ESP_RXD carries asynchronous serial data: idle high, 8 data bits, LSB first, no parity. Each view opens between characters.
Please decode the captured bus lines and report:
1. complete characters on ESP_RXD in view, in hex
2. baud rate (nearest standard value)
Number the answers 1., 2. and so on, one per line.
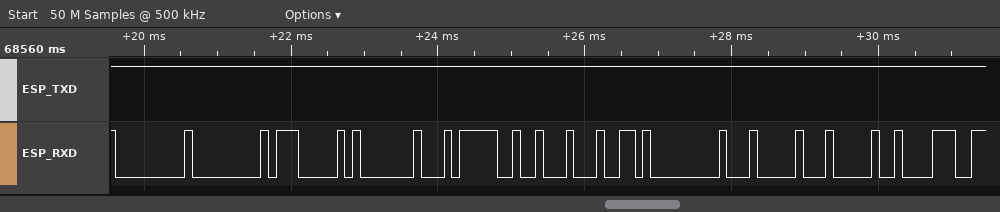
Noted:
1. 00, 00, 07, 01, F4, 12, 64, 00, 04, 04, C2
2. 9600 baud
